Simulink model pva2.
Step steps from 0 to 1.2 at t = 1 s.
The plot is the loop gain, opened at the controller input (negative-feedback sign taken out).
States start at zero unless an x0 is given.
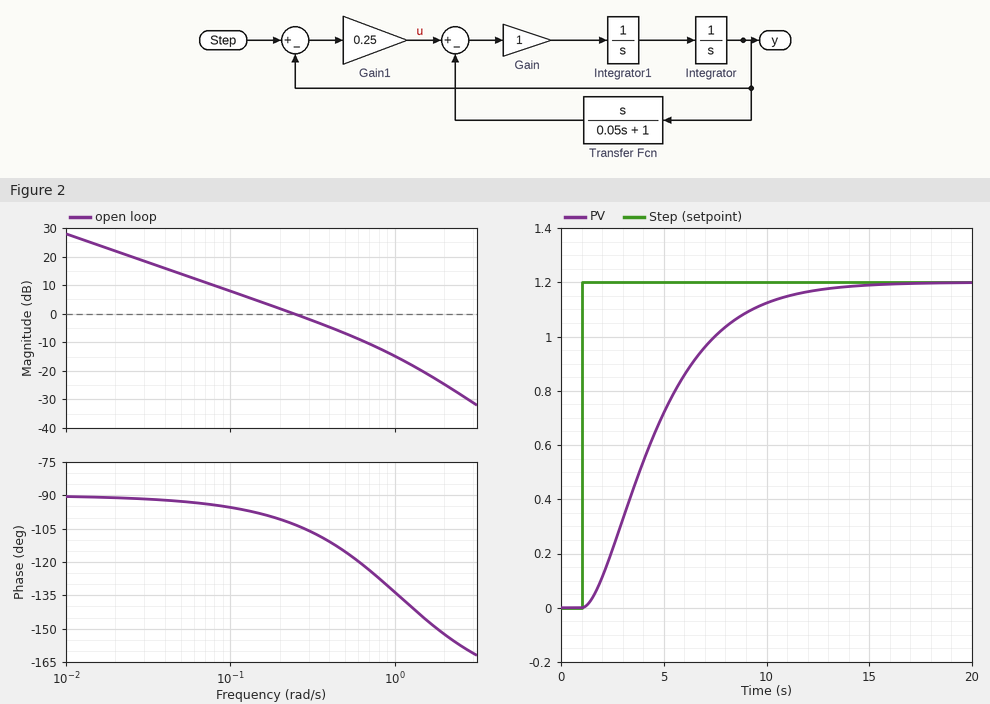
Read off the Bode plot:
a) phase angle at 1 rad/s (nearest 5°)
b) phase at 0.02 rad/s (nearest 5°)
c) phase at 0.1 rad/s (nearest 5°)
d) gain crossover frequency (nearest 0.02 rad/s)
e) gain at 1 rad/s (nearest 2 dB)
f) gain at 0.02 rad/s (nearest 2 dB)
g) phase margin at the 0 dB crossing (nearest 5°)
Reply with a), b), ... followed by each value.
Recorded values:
a) -135°
b) -90°
c) -95°
d) 0.24 rad/s
e) -14 dB
f) 22 dB
g) 75°
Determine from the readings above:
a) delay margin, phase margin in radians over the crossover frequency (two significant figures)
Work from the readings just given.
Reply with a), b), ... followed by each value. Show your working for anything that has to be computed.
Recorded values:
a) 75 × π / 180 / 0.24 = 5.5 s
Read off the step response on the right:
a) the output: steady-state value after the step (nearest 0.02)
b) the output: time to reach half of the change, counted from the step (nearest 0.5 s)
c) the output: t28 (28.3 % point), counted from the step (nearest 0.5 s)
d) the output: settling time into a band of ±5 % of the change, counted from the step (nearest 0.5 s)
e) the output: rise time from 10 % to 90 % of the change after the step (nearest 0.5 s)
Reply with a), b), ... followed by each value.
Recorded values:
a) 1.20
b) 3.5 s
c) 2.0 s
d) 9.5 s
e) 7.0 s
